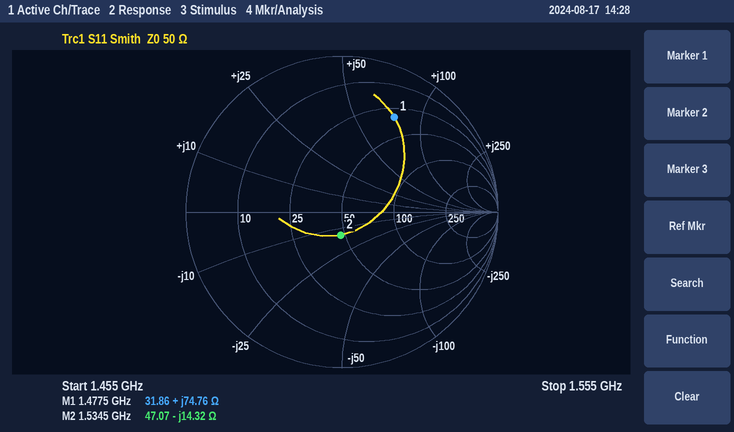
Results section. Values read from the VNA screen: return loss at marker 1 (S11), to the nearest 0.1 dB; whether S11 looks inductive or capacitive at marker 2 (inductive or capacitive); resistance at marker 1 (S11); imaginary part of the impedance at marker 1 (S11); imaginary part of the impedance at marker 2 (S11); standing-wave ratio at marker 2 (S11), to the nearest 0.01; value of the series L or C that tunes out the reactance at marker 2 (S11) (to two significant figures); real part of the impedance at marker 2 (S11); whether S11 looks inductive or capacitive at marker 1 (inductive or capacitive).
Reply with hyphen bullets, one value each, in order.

- 3.2 dB
- capacitive
- 31.86 Ω
- +74.76 Ω
- -14.32 Ω
- 1.35
- 1.5 nH
- 47.07 Ω
- inductive
